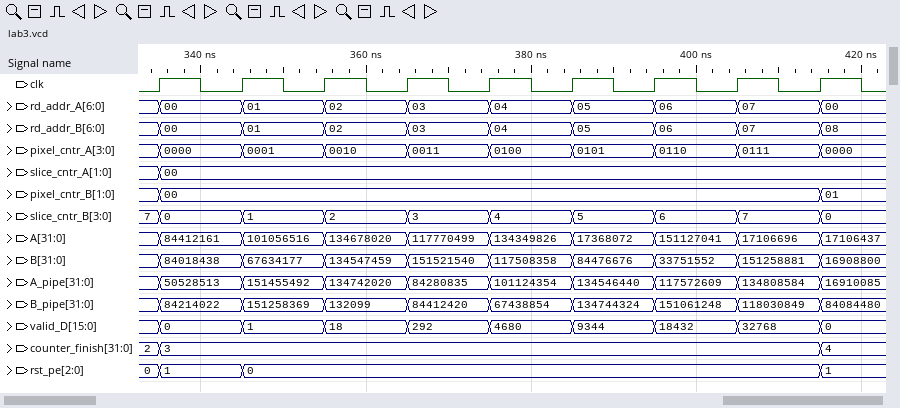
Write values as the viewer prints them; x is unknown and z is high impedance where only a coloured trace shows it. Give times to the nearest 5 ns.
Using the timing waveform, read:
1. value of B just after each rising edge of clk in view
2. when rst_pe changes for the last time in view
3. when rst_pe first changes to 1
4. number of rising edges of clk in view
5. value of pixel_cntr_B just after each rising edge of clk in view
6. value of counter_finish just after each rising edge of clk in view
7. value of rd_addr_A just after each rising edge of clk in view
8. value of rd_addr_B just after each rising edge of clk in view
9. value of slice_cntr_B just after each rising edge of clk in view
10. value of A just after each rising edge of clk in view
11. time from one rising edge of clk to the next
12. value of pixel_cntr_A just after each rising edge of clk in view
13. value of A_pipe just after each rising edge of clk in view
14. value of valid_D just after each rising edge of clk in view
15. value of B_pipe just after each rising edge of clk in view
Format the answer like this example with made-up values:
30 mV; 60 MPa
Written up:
84018438, 67634177, 134547459, 151521540, 117508358, 84476676, 33751552, 151258881, 16908800; 415 ns; 335 ns; 9; 00, 00, 00, 00, 00, 00, 00, 00, 01; 3, 3, 3, 3, 3, 3, 3, 3, 4; 00, 01, 02, 03, 04, 05, 06, 07, 00; 00, 01, 02, 03, 04, 05, 06, 07, 08; 0, 1, 2, 3, 4, 5, 6, 7, 0; 84412161, 101056516, 134678020, 117770499, 134349826, 17368072, 151127041, 17106696, 17106437; 10 ns; 0000, 0001, 0010, 0011, 0100, 0101, 0110, 0111, 0000; 50528513, 151455492, 134742020, 84280835, 101124354, 134546440, 117572609, 134808584, 16910085; 0, 1, 18, 292, 4680, 9344, 18432, 32768, 0; 84214022, 151258369, 132099, 84412420, 67438854, 134744324, 151061248, 118030849, 84084480
